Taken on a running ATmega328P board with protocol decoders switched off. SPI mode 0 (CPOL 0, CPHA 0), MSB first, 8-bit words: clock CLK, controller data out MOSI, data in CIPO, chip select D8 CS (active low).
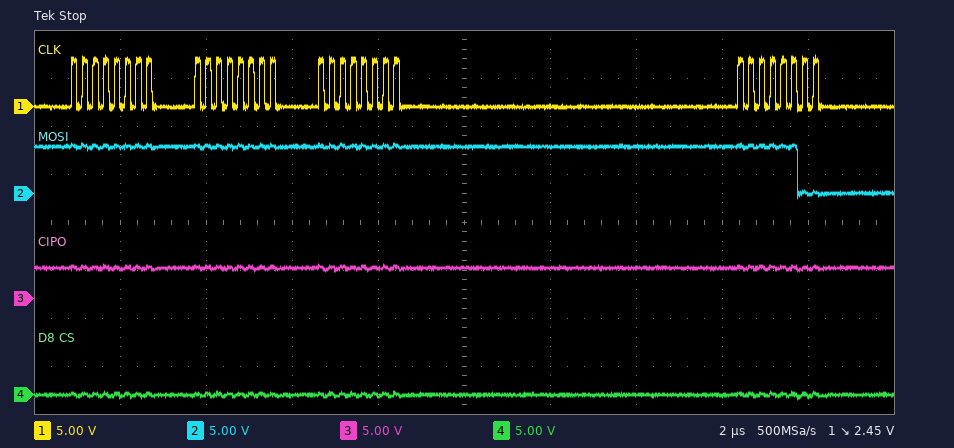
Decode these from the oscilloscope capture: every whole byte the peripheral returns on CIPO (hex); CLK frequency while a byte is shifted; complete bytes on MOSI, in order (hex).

FF FF FF FF
4 MHz
FF FF FF FC
